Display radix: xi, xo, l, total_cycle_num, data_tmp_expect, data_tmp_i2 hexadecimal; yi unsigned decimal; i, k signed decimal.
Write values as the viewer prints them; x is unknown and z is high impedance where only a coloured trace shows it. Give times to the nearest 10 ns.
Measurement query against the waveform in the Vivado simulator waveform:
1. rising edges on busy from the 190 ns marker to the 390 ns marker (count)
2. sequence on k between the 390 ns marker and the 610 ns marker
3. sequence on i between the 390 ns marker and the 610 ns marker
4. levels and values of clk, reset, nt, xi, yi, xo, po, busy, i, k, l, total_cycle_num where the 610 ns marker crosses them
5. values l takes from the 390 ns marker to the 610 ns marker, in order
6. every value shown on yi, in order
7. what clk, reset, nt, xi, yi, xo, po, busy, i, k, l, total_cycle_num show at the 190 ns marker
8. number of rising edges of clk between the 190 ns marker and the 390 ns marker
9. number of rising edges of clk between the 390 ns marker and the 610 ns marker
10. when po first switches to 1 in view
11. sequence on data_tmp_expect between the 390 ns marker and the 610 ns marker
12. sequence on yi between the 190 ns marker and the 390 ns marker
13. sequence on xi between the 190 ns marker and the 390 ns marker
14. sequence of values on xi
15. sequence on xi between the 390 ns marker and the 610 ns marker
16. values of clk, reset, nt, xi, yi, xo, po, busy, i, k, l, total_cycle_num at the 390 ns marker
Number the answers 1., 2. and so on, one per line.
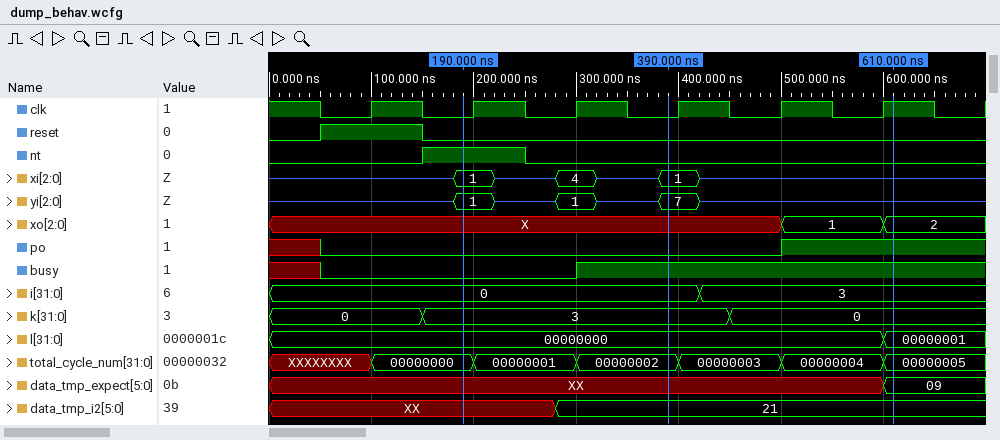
1. 1
2. 3, 0
3. 0, 3
4. clk=1, reset=0, nt=0, xi=z, yi=z, xo=2, po=1, busy=1, i=3, k=0, l=00000001, total_cycle_num=00000005
5. 00000000, 00000001
6. z, 1, z, 1, z, 7, z
7. clk=0, reset=0, nt=1, xi=1, yi=1, xo=X, po=0, busy=0, i=0, k=3, l=00000000, total_cycle_num=00000000
8. 2
9. 3
10. 500 ns
11. XX, 09
12. 1, z, 1, z, 7
13. 1, z, 4, z, 1
14. z, 1, z, 4, z, 1, z
15. 1, z
16. clk=0, reset=0, nt=0, xi=1, yi=7, xo=X, po=0, busy=1, i=0, k=3, l=00000000, total_cycle_num=00000002
